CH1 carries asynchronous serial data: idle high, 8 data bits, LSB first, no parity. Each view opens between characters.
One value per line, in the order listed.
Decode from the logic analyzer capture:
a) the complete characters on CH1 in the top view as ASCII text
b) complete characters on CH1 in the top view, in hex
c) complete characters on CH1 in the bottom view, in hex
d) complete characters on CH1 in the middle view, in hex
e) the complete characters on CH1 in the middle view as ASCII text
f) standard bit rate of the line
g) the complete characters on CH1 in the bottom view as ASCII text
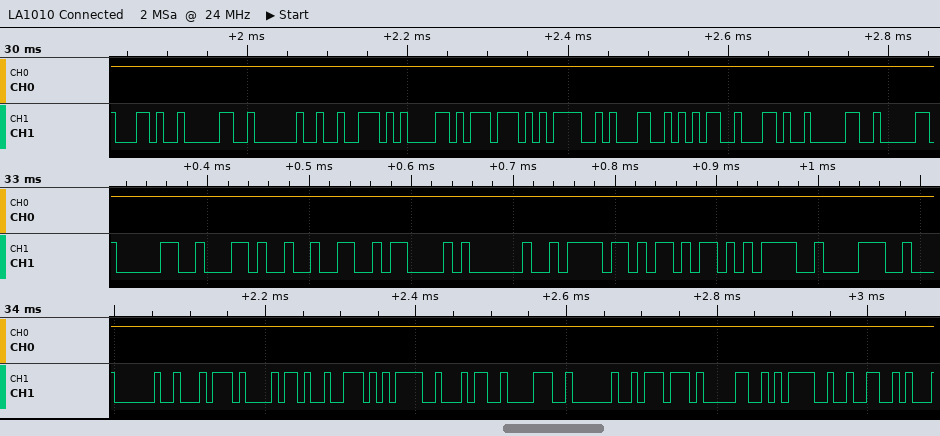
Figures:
",0 raw=15,0"
2C, 30, 20, 72, 61, 77, 3D, 31, 35, 2C, 30
20, 74, 68, 72, 3D, 34, 38, 20, 77, 30, 3D, 32
30, 2C, 32, 43, 20, 6F, 6B, 3D, 38
"0,2C ok=8"
115200 baud
" thr=48 w0=2"
